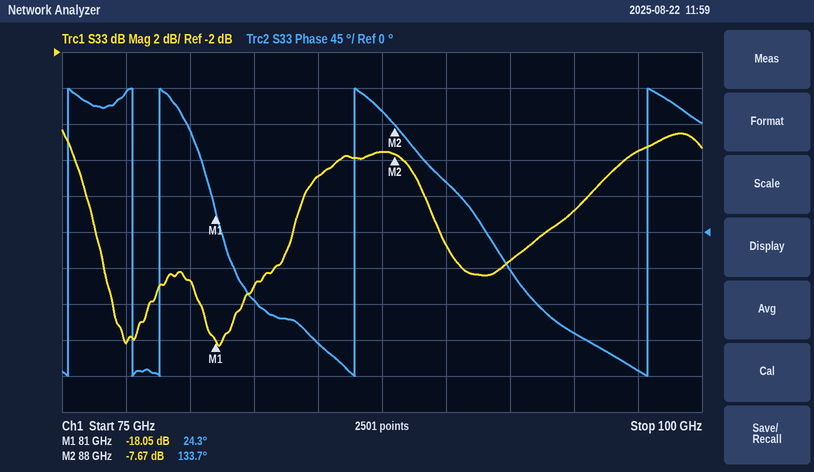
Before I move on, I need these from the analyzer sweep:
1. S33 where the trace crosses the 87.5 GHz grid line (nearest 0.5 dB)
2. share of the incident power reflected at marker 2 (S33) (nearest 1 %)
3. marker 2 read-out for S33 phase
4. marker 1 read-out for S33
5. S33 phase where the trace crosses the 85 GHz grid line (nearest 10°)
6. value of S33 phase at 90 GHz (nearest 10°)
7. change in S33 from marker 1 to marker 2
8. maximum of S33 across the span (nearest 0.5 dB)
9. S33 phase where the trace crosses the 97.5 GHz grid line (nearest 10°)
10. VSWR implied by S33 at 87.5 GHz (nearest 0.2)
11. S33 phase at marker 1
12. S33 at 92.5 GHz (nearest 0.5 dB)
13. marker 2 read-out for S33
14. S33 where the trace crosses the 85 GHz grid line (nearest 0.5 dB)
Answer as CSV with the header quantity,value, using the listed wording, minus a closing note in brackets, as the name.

quantity,value
S33 where the trace crosses the 87.5 GHz grid line,-7.5 dB
share of the incident power reflected at marker 2 (S33),17 %
marker 2 read-out for S33 phase,133.7°
marker 1 read-out for S33,-18.05 dB
S33 phase where the trace crosses the 85 GHz grid line,-140°
value of S33 phase at 90 GHz,60°
change in S33 from marker 1 to marker 2,10.38 dB
maximum of S33 across the span,-6.5 dB
S33 phase where the trace crosses the 97.5 GHz grid line,-170°
VSWR implied by S33 at 87.5 GHz,2.4
S33 phase at marker 1,24.3°
S33 at 92.5 GHz,-13.5 dB
marker 2 read-out for S33,-7.67 dB
S33 where the trace crosses the 85 GHz grid line,-9.0 dB
